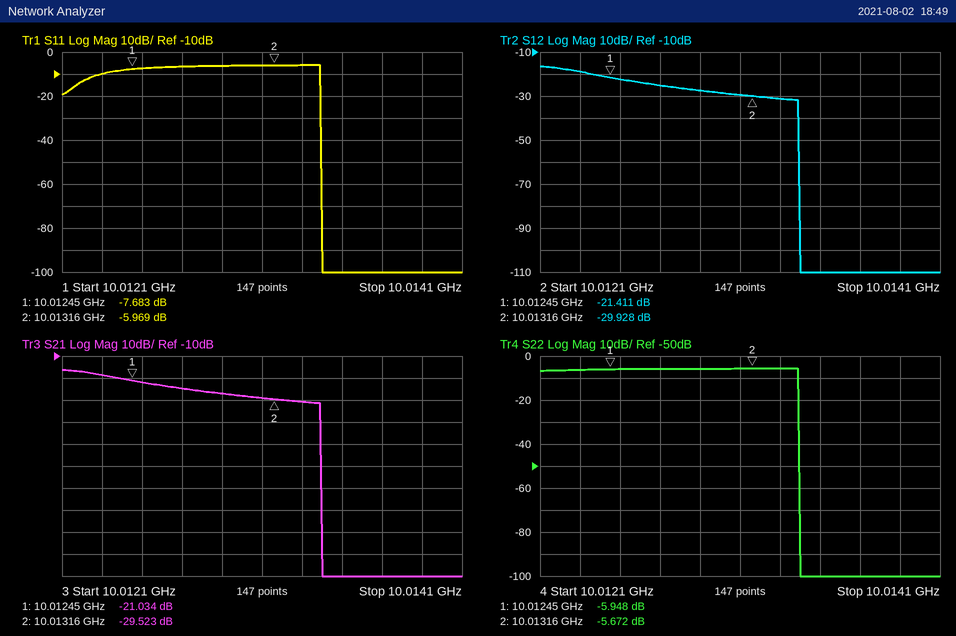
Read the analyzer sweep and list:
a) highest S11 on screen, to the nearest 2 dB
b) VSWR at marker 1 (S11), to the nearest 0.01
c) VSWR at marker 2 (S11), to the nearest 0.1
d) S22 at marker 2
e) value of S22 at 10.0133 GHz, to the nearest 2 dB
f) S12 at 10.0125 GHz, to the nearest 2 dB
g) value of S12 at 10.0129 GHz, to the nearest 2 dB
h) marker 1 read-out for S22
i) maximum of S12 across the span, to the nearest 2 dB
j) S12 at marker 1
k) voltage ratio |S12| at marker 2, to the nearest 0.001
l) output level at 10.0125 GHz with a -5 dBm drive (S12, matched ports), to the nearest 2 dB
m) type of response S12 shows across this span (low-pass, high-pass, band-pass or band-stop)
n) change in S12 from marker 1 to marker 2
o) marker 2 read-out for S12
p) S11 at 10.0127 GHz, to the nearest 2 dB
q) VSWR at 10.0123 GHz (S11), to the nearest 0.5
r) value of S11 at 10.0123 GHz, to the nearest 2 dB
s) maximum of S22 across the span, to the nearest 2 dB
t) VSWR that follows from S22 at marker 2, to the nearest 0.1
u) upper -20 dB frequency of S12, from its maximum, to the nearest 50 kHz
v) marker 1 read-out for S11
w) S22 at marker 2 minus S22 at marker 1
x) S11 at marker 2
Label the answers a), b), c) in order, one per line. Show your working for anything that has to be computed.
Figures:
a) -6 dB
b) (1 + 0.4129)/(1 − 0.4129) ≈ 2.41
c) (1 + 0.5030)/(1 − 0.5030) ≈ 3.0
d) -5.672 dB
e) -6 dB
f) -22 dB
g) -28 dB
h) -5.948 dB
i) -16 dB
j) -21.411 dB
k) 10^(-29.928/20) ≈ 0.032
l) -5 dBm + (-22 dB) = -28 dBm
m) low-pass
n) -29.928 − (-21.411) = -8.517 dB
o) -29.928 dB
p) -6 dB
q) |Γ| = 10^(-10/20) = 0.3162; VSWR = (1 + 0.3162)/(1 − 0.3162) ≈ 1.92, so 2.0 to the nearest 0.5
r) -10 dB
s) -6 dB
t) (1 + 0.5205)/(1 − 0.5205) ≈ 3.2
u) 10.01340 GHz
v) -7.683 dB
w) -5.672 − (-5.948) = 0.276 dB
x) -5.969 dB
